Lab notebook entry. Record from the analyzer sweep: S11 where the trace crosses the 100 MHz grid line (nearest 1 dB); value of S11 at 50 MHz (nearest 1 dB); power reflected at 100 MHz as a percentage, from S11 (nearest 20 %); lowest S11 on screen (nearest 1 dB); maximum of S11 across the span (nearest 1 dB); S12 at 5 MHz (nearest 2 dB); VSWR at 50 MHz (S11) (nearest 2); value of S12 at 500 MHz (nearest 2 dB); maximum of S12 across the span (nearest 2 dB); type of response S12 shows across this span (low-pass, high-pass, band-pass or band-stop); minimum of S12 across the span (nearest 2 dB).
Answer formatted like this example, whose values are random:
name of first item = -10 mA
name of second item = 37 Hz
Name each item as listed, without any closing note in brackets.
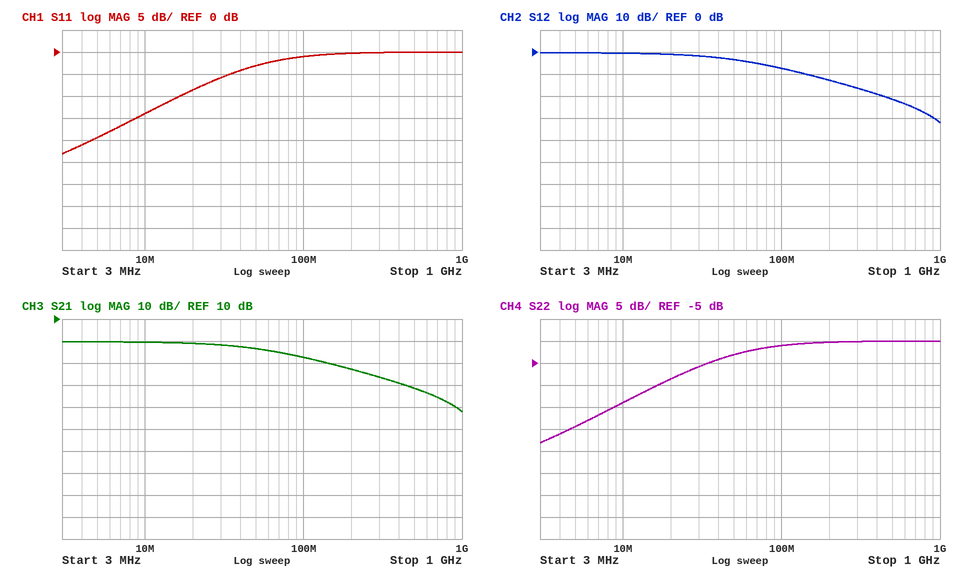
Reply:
S11 where the trace crosses the 100 MHz grid line = -1 dB
value of S11 at 50 MHz = -3 dB
power reflected at 100 MHz as a percentage, from S11 = 80 %
lowest S11 on screen = -23 dB
maximum of S11 across the span = 0 dB
S12 at 5 MHz = 0 dB
VSWR at 50 MHz (S11) = 6
value of S12 at 500 MHz = -22 dB
maximum of S12 across the span = 0 dB
type of response S12 shows across this span = low-pass
minimum of S12 across the span = -32 dB
